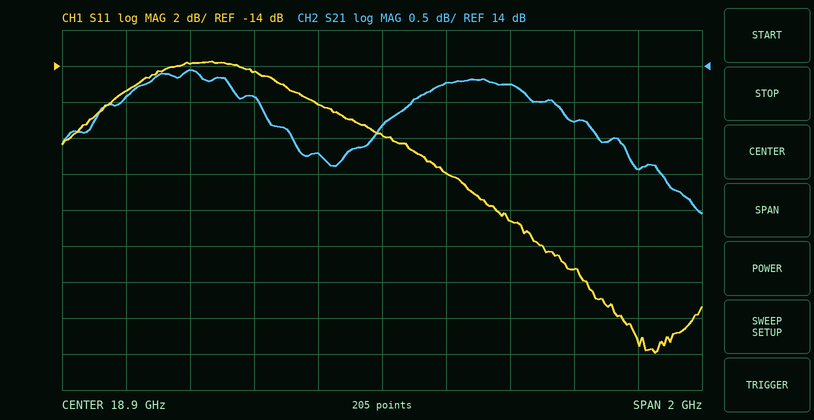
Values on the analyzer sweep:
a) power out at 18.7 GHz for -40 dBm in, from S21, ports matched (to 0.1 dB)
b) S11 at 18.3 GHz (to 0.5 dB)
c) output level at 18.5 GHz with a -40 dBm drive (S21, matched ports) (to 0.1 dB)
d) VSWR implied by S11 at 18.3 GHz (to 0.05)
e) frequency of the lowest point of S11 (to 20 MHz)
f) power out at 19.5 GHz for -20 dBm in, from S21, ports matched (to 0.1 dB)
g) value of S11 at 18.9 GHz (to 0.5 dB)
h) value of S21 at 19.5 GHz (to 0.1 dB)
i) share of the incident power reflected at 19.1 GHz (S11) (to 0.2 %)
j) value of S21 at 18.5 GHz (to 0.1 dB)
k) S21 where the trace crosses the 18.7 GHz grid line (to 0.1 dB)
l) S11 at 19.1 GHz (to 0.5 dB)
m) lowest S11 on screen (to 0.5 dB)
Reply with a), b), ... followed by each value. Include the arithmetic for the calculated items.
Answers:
a) -40 dBm + (12.8 dB) = -27.2 dBm
b) -14.0 dB
c) -40 dBm + (13.6 dB) = -26.4 dBm
d) |Γ| = 10^(-14/20) = 0.1995; VSWR = (1 + 0.1995)/(1 − 0.1995) ≈ 1.50
e) 19.76 GHz
f) -20 dBm + (13.2 dB) = -6.8 dBm
g) -18.0 dB
h) 13.2 dB
i) 10^(-20/10) ≈ 1.0 %
j) 13.6 dB
k) 12.8 dB
l) -20.0 dB
m) -30.0 dB
